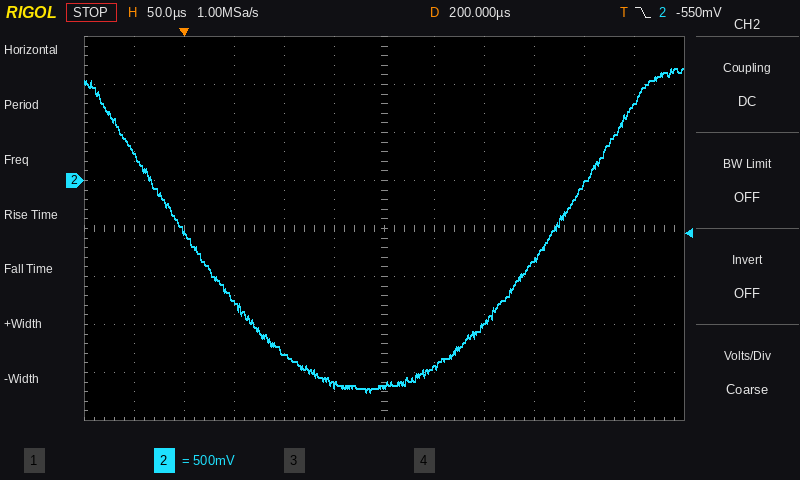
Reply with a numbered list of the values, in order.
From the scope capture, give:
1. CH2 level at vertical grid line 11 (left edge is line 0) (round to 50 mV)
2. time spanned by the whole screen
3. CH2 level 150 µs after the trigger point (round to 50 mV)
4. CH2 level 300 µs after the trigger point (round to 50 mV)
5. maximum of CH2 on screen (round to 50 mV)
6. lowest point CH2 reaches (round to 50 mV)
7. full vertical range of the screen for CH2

1. 800 mV
2. 600 µs
3. -2.15 V
4. -1.50 V
5. 1.15 V
6. -2.20 V
7. 4 V
